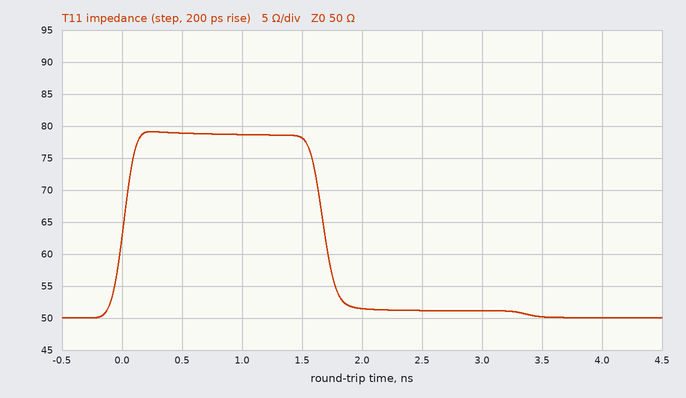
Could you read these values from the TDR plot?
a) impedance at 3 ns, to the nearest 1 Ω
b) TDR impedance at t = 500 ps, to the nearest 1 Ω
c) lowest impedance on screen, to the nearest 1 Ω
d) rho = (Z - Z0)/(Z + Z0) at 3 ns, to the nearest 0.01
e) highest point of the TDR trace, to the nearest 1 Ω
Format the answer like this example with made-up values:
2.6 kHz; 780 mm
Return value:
51 Ω; 79 Ω; 50 Ω; +0.01; 79 Ω
